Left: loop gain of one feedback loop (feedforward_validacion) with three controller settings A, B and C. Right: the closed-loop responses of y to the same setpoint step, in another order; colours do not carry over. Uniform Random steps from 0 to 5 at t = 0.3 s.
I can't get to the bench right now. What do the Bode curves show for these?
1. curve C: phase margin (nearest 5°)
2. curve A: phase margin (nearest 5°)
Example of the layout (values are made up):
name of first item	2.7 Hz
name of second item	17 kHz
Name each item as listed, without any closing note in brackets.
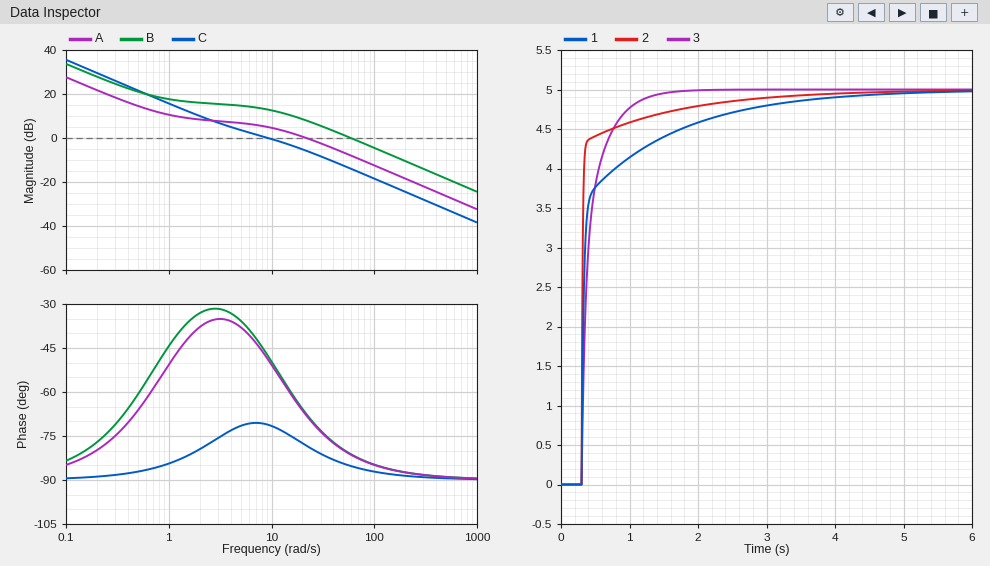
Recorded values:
curve C: phase margin	110°
curve A: phase margin	110°
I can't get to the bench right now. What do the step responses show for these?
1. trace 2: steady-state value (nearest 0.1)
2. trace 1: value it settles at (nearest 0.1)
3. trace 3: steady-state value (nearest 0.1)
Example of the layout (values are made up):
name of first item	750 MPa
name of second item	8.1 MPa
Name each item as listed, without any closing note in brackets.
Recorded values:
trace 2: steady-state value	5.0
trace 1: value it settles at	5.0
trace 3: steady-state value	5.0
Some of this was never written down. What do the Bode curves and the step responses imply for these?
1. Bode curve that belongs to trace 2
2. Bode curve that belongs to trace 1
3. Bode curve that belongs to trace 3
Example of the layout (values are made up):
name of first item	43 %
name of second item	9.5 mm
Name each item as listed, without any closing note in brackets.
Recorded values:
Bode curve that belongs to trace 2	B
Bode curve that belongs to trace 1	A
Bode curve that belongs to trace 3	C
